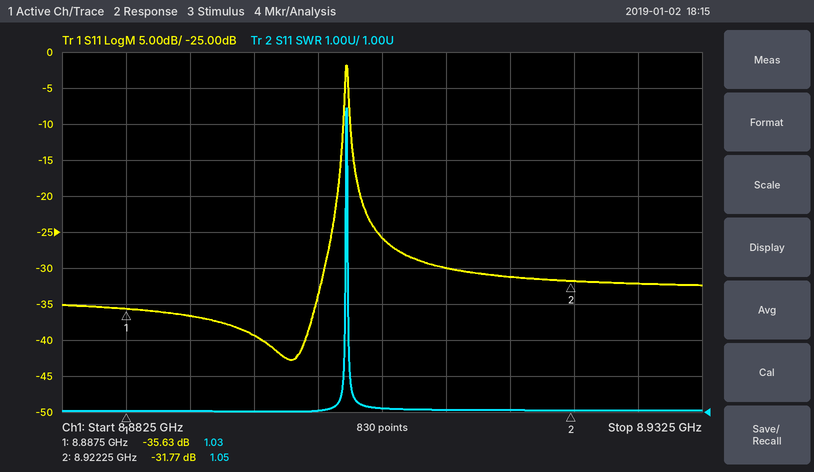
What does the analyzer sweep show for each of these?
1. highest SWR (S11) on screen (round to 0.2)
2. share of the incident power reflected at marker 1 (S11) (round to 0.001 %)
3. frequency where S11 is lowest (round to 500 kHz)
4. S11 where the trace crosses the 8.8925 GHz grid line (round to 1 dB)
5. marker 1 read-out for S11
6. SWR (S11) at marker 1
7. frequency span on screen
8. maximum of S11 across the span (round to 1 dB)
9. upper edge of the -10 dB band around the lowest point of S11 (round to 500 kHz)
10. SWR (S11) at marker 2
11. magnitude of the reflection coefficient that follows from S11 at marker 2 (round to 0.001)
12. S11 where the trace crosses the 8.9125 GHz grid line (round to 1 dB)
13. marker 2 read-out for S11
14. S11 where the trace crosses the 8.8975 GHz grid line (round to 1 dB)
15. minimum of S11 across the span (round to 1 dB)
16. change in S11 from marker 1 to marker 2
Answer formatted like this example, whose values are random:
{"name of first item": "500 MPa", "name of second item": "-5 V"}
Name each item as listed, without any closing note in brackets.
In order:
{"highest SWR (S11) on screen": "9.4", "share of the incident power reflected at marker 1 (S11)": "0.027 %", "frequency where S11 is lowest": "8.9005 GHz", "S11 where the trace crosses the 8.8925 GHz grid line": "-37 dB", "marker 1 read-out for S11": "-35.63 dB", "SWR (S11) at marker 1": "1.03", "frequency span on screen": "50 MHz", "maximum of S11 across the span": "-2 dB", "upper edge of the -10 dB band around the lowest point of S11": "8.9045 GHz", "SWR (S11) at marker 2": "1.05", "magnitude of the reflection coefficient that follows from S11 at marker 2": "0.026", "S11 where the trace crosses the 8.9125 GHz grid line": "-30 dB", "marker 2 read-out for S11": "-31.77 dB", "S11 where the trace crosses the 8.8975 GHz grid line": "-39 dB", "minimum of S11 across the span": "-43 dB", "change in S11 from marker 1 to marker 2": "3.86 dB"}
